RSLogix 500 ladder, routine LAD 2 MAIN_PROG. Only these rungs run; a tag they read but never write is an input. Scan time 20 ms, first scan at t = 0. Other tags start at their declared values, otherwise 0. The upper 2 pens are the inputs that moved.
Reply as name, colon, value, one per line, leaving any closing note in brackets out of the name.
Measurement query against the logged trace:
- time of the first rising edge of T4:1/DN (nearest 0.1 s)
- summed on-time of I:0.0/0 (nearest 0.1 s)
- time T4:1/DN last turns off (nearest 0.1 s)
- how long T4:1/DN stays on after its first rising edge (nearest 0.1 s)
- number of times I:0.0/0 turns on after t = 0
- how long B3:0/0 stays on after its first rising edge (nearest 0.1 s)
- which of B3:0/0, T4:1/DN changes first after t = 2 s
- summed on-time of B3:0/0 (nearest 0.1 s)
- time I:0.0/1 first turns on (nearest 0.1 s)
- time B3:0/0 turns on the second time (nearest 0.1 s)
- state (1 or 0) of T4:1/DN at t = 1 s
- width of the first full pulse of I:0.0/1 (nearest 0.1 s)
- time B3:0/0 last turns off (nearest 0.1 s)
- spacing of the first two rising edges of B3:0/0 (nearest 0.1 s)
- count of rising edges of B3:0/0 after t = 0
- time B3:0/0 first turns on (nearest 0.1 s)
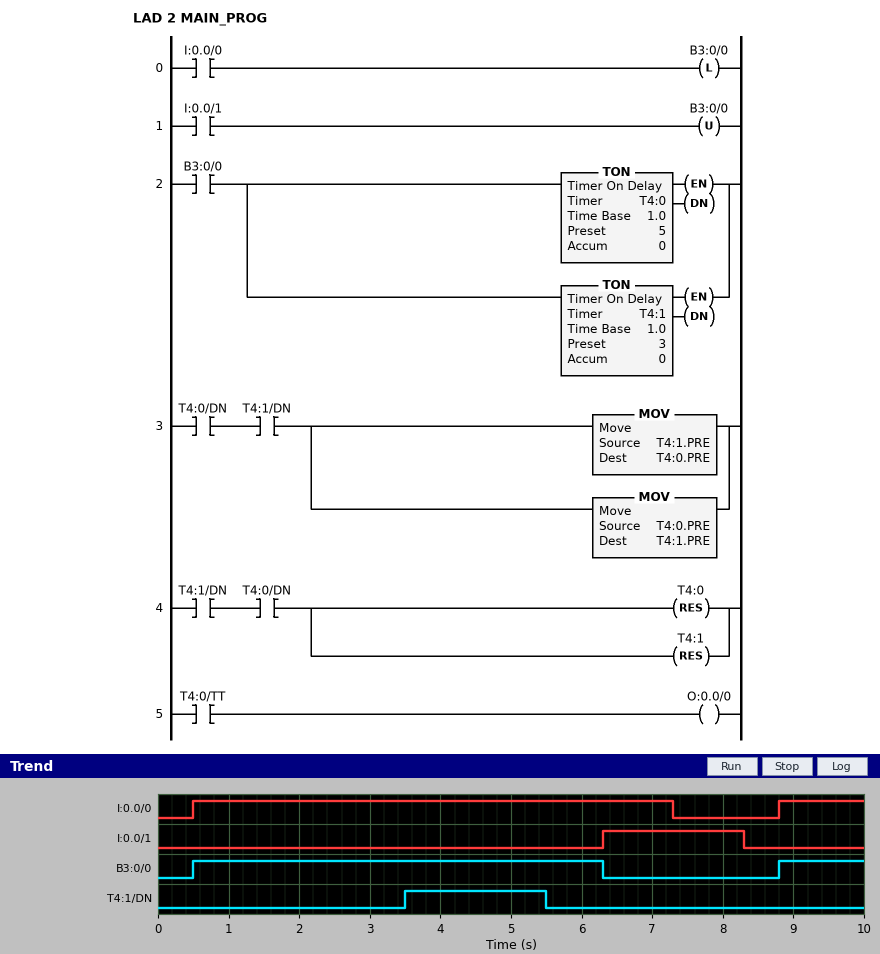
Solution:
time of the first rising edge of T4:1/DN: 3.5 s
summed on-time of I:0.0/0: 8.0 s
time T4:1/DN last turns off: 5.5 s
how long T4:1/DN stays on after its first rising edge: 2.0 s
number of times I:0.0/0 turns on after t = 0: 2
how long B3:0/0 stays on after its first rising edge: 5.8 s
which of B3:0/0, T4:1/DN changes first after t = 2 s: T4:1/DN
summed on-time of B3:0/0: 7.0 s
time I:0.0/1 first turns on: 6.3 s
time B3:0/0 turns on the second time: 8.8 s
state (1 or 0) of T4:1/DN at t = 1 s: 0
width of the first full pulse of I:0.0/1: 2.0 s
time B3:0/0 last turns off: 6.3 s
spacing of the first two rising edges of B3:0/0: 8.3 s
count of rising edges of B3:0/0 after t = 0: 2
time B3:0/0 first turns on: 0.5 s
